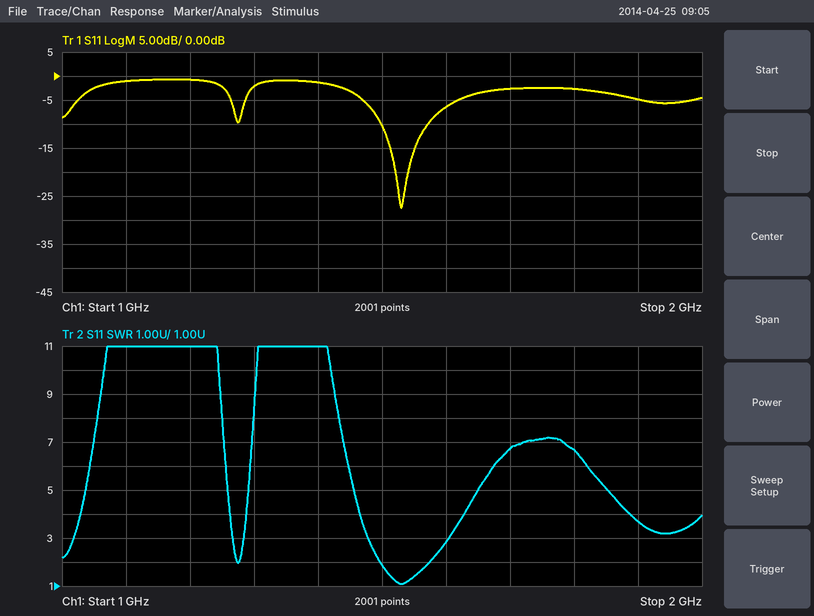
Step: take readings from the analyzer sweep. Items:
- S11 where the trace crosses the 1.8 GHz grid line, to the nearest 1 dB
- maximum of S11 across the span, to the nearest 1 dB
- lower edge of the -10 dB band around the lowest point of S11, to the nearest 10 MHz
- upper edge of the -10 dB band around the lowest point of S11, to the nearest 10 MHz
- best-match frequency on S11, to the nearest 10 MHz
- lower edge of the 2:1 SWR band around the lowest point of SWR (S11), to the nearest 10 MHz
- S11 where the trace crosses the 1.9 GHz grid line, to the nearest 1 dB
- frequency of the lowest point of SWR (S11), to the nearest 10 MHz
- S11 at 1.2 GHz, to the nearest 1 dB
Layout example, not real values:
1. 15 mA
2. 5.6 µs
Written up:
1. -3 dB
2. -1 dB
3. 1.50 GHz
4. 1.57 GHz
5. 1.53 GHz
6. 1.50 GHz
7. -5 dB
8. 1.53 GHz
9. -1 dB
